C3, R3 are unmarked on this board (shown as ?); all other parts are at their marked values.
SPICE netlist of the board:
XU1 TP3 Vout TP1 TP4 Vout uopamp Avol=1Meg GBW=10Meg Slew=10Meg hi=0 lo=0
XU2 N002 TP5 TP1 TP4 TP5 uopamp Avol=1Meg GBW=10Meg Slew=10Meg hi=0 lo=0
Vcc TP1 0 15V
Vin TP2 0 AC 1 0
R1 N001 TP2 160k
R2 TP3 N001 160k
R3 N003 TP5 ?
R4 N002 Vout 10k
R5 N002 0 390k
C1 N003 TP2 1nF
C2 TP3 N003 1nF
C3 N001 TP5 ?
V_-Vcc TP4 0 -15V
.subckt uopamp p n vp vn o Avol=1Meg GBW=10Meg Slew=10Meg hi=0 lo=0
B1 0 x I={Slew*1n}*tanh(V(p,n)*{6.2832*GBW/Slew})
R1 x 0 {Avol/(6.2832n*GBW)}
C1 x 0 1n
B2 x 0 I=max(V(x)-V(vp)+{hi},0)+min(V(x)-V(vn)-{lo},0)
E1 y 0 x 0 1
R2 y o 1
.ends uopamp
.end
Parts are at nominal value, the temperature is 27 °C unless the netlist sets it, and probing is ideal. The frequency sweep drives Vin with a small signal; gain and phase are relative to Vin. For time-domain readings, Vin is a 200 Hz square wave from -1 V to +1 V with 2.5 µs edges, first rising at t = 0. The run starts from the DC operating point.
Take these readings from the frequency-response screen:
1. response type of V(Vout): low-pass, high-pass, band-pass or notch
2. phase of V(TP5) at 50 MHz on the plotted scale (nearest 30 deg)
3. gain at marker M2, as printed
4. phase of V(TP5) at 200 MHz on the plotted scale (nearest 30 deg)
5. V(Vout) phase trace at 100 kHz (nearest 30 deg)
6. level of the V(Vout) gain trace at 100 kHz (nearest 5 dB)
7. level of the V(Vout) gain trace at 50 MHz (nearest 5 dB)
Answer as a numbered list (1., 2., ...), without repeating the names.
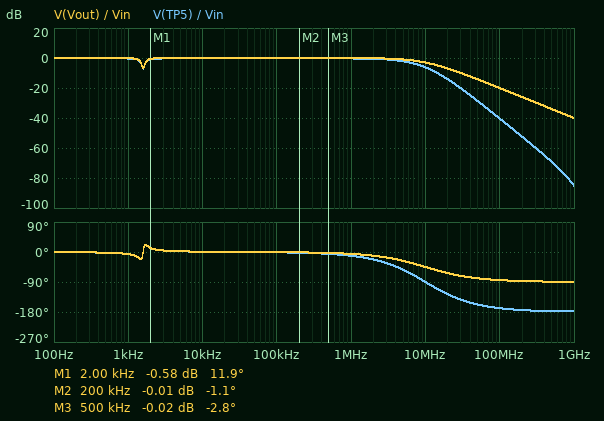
1. low-pass
2. -150 deg
3. -0.01 dB
4. -180 deg
5. 0 deg
6. 0 dB
7. -15 dB
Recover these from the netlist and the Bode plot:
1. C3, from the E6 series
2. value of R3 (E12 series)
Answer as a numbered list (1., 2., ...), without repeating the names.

1. 680 pF
2. 33 kΩ
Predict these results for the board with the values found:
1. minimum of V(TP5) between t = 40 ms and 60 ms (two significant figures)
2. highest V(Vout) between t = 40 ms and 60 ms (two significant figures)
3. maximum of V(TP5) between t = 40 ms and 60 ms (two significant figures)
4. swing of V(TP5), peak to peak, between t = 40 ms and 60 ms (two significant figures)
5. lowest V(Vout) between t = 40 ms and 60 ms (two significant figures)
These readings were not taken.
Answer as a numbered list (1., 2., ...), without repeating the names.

1. -1.1 V
2. 1.1 V
3. 1.1 V
4. 2.2 V
5. -1.1 V
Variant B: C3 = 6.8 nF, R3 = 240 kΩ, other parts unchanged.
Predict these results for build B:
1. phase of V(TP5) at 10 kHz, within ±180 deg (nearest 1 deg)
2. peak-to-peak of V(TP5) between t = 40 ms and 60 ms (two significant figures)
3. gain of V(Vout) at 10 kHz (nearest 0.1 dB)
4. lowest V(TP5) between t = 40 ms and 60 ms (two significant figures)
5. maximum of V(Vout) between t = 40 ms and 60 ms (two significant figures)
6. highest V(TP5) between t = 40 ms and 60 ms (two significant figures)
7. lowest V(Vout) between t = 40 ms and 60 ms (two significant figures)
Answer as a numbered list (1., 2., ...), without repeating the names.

1. 0 deg
2. 2.5 V
3. 0 dB
4. -1.2 V
5. 1.3 V
6. 1.2 V
7. -1.3 V
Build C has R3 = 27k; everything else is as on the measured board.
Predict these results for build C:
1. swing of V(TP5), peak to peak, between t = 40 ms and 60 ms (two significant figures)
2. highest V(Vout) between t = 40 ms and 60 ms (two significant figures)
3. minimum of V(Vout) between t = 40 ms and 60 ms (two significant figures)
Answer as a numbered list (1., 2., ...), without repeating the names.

1. 2.3 V
2. 1.2 V
3. -1.2 V
